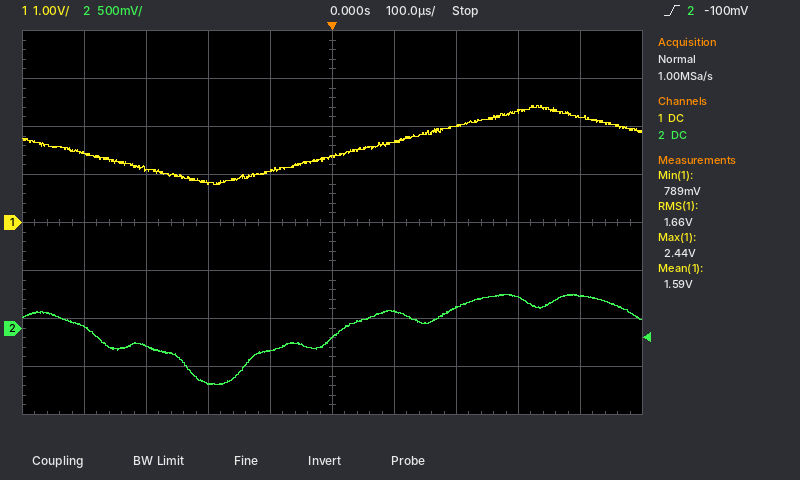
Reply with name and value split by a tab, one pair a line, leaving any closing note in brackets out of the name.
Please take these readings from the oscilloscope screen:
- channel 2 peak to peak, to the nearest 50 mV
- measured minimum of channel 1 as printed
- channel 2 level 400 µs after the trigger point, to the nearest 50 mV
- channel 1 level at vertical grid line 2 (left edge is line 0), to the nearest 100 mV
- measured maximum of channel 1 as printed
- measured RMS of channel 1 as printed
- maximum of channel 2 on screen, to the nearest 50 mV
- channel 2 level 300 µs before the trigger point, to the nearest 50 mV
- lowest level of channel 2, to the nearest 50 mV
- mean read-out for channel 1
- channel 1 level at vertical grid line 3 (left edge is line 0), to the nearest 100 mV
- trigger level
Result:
channel 2 peak to peak, to the nearest 50 mV	950 mV
measured minimum of channel 1 as printed	789 mV
channel 2 level 400 µs after the trigger point, to the nearest 50 mV	350 mV
channel 1 level at vertical grid line 2 (left edge is line 0), to the nearest 100 mV	1.1 V
measured maximum of channel 1 as printed	2.44 V
measured RMS of channel 1 as printed	1.66 V
maximum of channel 2 on screen, to the nearest 50 mV	350 mV
channel 2 level 300 µs before the trigger point, to the nearest 50 mV	-200 mV
lowest level of channel 2, to the nearest 50 mV	-600 mV
mean read-out for channel 1	1.59 V
channel 1 level at vertical grid line 3 (left edge is line 0), to the nearest 100 mV	800 mV
trigger level	-100 mV
